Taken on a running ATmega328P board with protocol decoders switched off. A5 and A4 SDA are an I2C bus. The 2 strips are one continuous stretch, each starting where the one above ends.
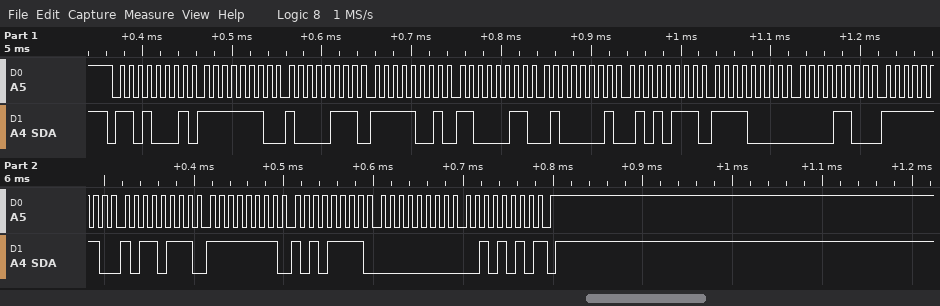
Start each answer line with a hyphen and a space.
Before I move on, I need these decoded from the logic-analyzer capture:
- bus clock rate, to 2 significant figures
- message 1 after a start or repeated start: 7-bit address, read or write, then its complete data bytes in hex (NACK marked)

- 100 kHz
- 0x68 read: FE 87 F9 C3 41 57 F0 0C FE B7 FF AF 00 2A NACK
